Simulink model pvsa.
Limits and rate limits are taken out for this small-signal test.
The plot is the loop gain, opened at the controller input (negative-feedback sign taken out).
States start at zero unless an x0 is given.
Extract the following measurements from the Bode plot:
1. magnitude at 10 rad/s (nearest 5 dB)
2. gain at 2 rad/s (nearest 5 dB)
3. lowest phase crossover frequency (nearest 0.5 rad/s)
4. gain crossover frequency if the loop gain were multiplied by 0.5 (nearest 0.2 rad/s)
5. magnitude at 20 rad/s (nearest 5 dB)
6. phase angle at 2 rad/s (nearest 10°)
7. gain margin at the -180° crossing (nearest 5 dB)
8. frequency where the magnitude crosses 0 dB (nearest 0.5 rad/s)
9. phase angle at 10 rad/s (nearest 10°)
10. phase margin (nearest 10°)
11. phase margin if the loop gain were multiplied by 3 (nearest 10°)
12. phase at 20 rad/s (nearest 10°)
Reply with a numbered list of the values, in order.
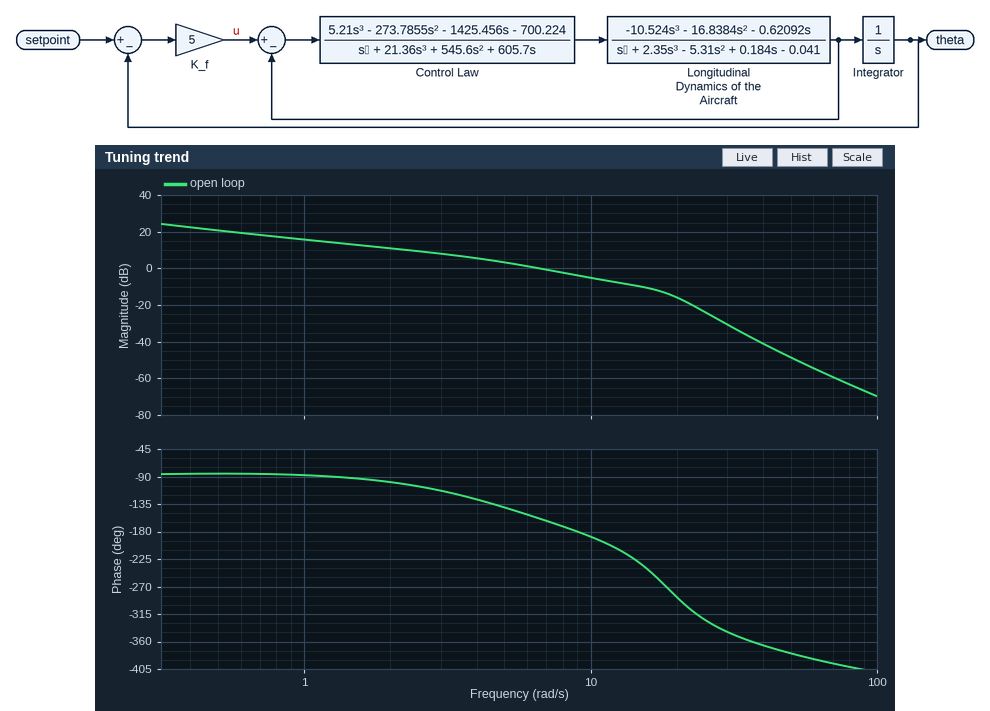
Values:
1. -5 dB
2. 10 dB
3. 9.0 rad/s
4. 3.8 rad/s
5. -15 dB
6. -100°
7. 5 dB
8. 6.5 rad/s
9. -190°
10. 20°
11. -50°
12. -290°
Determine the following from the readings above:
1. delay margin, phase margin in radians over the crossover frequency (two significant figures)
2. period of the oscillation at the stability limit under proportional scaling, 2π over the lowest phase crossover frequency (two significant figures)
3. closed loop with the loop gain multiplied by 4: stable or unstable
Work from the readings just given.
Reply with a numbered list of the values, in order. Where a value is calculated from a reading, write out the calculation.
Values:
1. 20 × π / 180 / 6.5 = 0.054 s
2. 2π / 9 = 0.70 s
3. unstable
